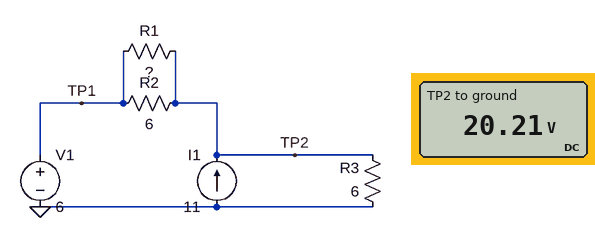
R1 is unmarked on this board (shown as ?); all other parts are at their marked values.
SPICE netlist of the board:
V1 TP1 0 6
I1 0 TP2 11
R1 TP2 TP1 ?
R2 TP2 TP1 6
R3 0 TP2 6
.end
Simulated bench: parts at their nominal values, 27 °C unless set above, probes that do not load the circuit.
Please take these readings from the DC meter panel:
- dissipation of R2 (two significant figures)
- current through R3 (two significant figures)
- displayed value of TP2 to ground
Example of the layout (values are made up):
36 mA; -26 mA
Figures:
34 W; 3.4 A; 20.21 V
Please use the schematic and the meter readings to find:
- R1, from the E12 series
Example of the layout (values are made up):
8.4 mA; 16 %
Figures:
2.7 Ω
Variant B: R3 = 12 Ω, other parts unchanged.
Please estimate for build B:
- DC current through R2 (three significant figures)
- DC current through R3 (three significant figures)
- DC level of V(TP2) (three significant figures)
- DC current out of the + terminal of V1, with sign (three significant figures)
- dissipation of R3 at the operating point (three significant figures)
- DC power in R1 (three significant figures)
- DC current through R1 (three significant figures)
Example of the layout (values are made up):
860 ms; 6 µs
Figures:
2.82 A; 1.91 A; 22.9 V; -9.09 A; 43.8 W; 106 W; 6.27 A
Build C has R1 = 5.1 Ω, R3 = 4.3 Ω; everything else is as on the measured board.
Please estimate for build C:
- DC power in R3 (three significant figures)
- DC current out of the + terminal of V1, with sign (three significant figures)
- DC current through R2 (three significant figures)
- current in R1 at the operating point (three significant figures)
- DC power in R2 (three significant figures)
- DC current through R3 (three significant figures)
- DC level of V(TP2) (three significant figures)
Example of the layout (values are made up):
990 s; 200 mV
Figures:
114 W; -5.85 A; 2.69 A; 3.16 A; 43.4 W; 5.15 A; 22.1 V
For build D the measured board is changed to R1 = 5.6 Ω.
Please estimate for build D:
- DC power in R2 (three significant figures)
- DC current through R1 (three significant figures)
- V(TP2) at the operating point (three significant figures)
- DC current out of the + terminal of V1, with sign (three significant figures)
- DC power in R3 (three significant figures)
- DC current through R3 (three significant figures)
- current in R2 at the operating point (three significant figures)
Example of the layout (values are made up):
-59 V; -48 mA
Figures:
63.6 W; 3.49 A; 25.5 V; -6.74 A; 109 W; 4.26 A; 3.26 A
